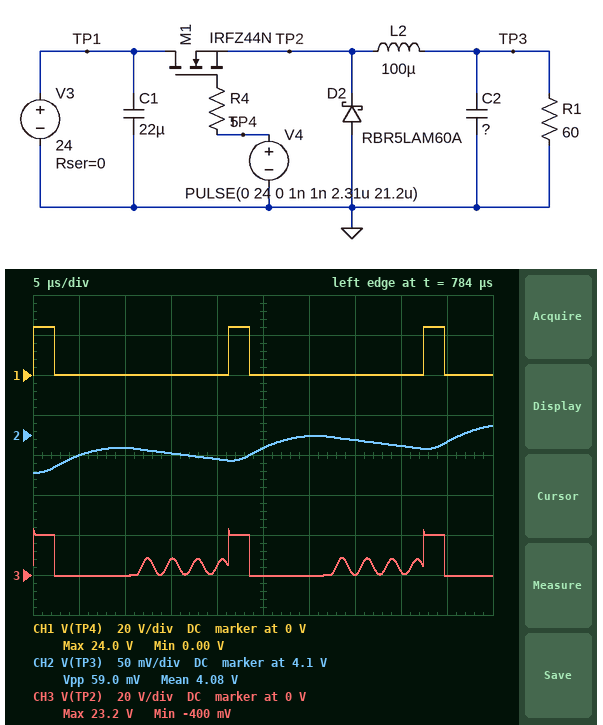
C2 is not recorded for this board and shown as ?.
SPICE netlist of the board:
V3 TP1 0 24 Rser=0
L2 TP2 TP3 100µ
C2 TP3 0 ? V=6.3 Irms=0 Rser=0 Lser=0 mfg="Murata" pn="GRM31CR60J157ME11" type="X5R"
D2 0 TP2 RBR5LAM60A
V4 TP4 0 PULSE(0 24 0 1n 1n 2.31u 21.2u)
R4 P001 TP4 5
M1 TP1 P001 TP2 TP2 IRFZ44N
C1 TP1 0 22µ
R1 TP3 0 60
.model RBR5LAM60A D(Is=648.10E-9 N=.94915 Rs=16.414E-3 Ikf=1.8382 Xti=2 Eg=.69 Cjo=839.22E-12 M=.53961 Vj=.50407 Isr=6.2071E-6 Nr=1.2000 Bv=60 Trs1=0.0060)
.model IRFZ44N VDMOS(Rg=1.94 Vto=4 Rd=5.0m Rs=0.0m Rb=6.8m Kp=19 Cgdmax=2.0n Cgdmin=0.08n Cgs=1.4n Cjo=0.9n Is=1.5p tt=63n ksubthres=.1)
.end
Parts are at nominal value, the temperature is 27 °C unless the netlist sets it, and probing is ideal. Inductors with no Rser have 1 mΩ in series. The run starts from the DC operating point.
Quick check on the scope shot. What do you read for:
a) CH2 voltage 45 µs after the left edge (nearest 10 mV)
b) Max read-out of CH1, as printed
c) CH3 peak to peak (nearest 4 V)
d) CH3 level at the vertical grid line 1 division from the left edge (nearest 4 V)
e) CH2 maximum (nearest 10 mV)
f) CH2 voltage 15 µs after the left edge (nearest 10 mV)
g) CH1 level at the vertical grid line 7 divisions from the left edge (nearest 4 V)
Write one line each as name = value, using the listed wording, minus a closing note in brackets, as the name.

CH2 voltage 45 µs after the left edge = 4.09 V
Max read-out of CH1, as printed = 24.0 V
CH3 peak to peak = 24 V
CH3 level at the vertical grid line 1 division from the left edge = 0 V
CH2 maximum = 4.11 V
CH2 voltage 15 µs after the left edge = 4.08 V
CH1 level at the vertical grid line 7 divisions from the left edge = 0 V
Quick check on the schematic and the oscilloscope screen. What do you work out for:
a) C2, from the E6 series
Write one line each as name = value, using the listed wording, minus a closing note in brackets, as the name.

C2, from the E6 series = 47 µF
